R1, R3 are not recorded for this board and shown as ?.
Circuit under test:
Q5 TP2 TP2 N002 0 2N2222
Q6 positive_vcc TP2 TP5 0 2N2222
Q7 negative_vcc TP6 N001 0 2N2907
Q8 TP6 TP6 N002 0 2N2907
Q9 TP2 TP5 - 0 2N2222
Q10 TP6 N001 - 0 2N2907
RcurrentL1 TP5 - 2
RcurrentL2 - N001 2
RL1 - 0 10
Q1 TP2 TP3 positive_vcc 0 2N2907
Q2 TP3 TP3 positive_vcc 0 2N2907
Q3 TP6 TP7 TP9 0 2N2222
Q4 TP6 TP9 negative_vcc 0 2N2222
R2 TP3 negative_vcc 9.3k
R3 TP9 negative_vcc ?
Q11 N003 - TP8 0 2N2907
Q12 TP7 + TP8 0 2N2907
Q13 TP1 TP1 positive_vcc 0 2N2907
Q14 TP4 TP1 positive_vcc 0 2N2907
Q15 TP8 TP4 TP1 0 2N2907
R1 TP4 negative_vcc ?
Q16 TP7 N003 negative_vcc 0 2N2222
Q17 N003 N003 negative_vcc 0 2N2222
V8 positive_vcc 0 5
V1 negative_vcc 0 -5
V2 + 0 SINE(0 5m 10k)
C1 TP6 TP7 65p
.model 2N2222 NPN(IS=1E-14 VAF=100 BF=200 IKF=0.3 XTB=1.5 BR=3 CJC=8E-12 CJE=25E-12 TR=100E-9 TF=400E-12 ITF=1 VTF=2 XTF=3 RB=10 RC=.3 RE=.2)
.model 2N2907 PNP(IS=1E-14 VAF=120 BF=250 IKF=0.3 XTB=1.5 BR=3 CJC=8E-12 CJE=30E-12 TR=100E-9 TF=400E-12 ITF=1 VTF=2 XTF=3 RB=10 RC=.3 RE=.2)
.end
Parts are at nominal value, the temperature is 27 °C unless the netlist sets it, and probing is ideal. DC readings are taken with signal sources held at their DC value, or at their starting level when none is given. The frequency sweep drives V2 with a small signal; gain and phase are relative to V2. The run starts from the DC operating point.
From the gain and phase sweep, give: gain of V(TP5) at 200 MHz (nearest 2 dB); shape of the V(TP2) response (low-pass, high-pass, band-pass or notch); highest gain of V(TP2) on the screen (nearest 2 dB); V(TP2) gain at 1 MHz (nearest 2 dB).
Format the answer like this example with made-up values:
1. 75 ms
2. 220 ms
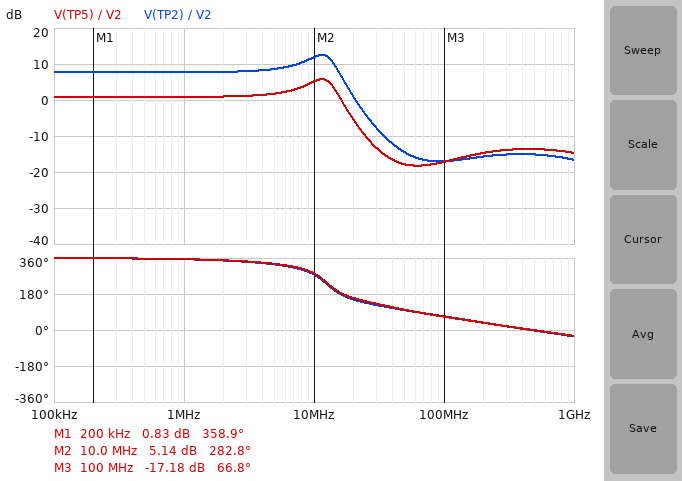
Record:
1. -14 dB
2. low-pass
3. 12 dB
4. 8 dB
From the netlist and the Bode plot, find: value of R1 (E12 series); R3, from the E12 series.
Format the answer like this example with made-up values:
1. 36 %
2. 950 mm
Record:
1. 15 kΩ
2. 4.7 kΩ
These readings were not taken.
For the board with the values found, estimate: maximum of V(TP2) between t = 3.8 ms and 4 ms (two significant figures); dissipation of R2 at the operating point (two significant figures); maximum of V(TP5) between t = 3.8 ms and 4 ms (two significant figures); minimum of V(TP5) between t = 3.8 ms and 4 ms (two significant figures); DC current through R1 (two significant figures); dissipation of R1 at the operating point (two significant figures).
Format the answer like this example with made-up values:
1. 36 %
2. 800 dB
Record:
1. 670 mV
2. 9.4 mW
3. 7.6 mV
4. -3.4 mV
5. 580 µA
6. 5.1 mW
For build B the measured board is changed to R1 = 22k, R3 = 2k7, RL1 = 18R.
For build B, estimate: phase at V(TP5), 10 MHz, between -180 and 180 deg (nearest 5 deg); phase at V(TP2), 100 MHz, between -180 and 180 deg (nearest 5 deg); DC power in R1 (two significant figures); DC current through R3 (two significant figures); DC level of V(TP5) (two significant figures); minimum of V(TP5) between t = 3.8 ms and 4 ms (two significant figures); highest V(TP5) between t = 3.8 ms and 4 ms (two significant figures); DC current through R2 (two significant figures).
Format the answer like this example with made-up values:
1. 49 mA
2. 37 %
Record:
1. -90 deg
2. 60 deg
3. 3.5 mW
4. 240 µA
5. 2.2 mV
6. -3.1 mV
7. 7.5 mV
8. 1.0 mA
